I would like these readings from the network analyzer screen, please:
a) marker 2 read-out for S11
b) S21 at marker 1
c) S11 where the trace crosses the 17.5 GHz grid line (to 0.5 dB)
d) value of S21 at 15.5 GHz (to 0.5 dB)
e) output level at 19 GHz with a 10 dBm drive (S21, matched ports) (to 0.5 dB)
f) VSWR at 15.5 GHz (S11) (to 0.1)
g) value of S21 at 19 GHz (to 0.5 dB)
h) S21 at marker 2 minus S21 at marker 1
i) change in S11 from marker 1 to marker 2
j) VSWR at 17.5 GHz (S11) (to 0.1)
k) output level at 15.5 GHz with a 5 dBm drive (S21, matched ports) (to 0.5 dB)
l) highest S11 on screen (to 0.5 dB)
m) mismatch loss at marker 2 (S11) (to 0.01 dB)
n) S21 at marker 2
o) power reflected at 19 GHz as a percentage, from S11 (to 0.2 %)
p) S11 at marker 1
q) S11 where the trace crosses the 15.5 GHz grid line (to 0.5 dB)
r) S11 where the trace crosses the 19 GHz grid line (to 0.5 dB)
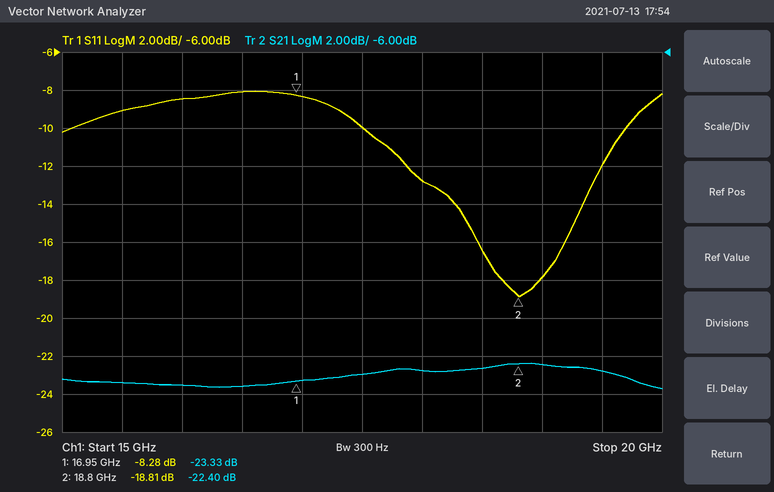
-18.81 dB
-23.33 dB
-10.0 dB
-23.5 dB
-12.5 dBm
2.1
-22.5 dB
0.93 dB
-10.53 dB
1.9
-18.5 dBm
-8.0 dB
0.06 dB
-22.40 dB
1.6 %
-8.28 dB
-9.0 dB
-18.0 dB
